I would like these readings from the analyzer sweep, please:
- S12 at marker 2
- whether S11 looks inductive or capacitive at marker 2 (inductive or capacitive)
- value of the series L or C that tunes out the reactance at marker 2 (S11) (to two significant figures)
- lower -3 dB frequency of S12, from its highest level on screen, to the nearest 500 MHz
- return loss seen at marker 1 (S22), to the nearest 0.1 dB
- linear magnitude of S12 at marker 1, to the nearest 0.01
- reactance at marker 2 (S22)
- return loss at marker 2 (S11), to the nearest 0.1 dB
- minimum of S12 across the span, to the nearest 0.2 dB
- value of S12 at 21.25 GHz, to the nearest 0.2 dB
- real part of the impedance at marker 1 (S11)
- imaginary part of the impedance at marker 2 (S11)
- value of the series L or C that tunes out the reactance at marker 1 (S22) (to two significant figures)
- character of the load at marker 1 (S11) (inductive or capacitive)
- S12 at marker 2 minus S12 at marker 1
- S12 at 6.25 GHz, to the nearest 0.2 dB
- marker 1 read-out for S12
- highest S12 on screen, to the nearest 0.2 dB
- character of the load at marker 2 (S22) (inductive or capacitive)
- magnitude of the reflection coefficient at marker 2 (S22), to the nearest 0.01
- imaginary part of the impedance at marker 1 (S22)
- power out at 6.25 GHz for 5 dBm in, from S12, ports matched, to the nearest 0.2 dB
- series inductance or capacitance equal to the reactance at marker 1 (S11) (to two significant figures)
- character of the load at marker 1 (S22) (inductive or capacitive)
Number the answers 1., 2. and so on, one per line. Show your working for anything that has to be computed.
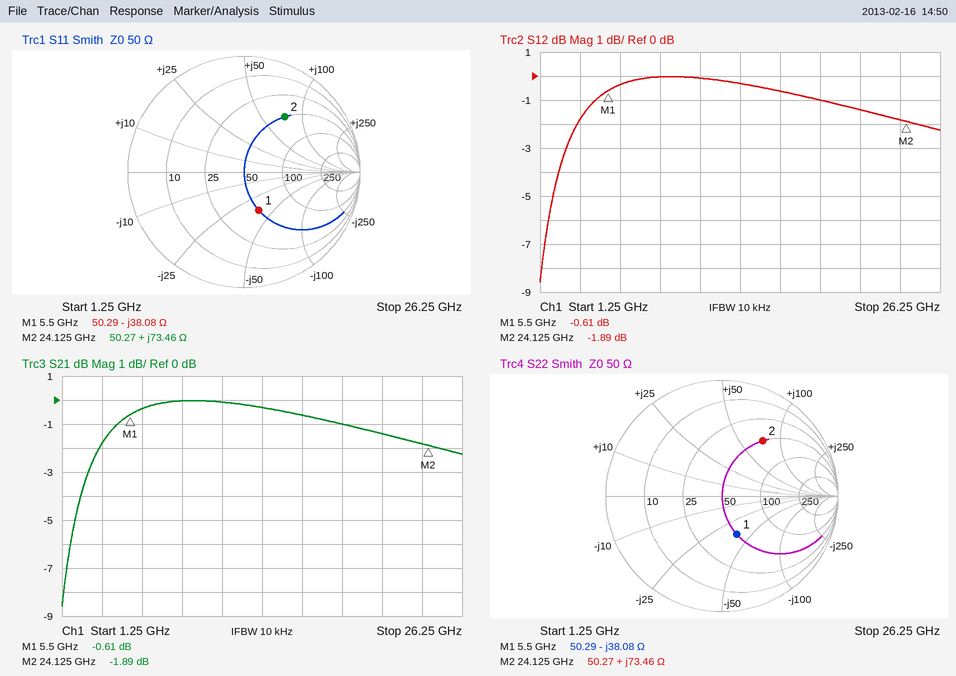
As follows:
1. -1.89 dB
2. inductive
3. C = 1/(2π × 24.125 GHz × 73.46 Ω) ≈ 90 fF
4. 3.0 GHz
5. 9.0 dB
6. 10^(-0.61/20) ≈ 0.93
7. +73.46 Ω
8. 4.6 dB
9. -8.6 dB
10. -1.4 dB
11. 50.29 Ω
12. +73.46 Ω
13. L = 38.08 Ω/(2π × 5.5 GHz) ≈ 1.1 nH
14. capacitive
15. -1.89 − (-0.61) = -1.28 dB
16. -0.4 dB
17. -0.61 dB
18. 0.0 dB
19. inductive
20. 0.59
21. -38.08 Ω
22. 5 dBm + (-0.4 dB) = 4.6 dBm
23. C = 1/(2π × 5.5 GHz × 38.08 Ω) ≈ 760 fF
24. capacitive
